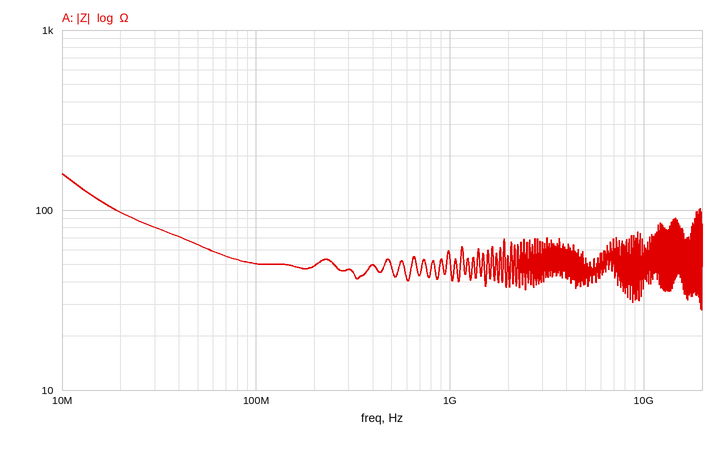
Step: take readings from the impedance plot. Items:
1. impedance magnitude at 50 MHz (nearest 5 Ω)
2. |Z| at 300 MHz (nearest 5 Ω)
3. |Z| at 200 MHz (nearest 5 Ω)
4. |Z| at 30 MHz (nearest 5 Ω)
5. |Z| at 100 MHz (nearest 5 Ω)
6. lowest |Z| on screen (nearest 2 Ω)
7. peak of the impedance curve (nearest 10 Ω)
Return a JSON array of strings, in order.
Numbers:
["65 Ω", "45 Ω", "50 Ω", "80 Ω", "50 Ω", "28 Ω", "160 Ω"]
